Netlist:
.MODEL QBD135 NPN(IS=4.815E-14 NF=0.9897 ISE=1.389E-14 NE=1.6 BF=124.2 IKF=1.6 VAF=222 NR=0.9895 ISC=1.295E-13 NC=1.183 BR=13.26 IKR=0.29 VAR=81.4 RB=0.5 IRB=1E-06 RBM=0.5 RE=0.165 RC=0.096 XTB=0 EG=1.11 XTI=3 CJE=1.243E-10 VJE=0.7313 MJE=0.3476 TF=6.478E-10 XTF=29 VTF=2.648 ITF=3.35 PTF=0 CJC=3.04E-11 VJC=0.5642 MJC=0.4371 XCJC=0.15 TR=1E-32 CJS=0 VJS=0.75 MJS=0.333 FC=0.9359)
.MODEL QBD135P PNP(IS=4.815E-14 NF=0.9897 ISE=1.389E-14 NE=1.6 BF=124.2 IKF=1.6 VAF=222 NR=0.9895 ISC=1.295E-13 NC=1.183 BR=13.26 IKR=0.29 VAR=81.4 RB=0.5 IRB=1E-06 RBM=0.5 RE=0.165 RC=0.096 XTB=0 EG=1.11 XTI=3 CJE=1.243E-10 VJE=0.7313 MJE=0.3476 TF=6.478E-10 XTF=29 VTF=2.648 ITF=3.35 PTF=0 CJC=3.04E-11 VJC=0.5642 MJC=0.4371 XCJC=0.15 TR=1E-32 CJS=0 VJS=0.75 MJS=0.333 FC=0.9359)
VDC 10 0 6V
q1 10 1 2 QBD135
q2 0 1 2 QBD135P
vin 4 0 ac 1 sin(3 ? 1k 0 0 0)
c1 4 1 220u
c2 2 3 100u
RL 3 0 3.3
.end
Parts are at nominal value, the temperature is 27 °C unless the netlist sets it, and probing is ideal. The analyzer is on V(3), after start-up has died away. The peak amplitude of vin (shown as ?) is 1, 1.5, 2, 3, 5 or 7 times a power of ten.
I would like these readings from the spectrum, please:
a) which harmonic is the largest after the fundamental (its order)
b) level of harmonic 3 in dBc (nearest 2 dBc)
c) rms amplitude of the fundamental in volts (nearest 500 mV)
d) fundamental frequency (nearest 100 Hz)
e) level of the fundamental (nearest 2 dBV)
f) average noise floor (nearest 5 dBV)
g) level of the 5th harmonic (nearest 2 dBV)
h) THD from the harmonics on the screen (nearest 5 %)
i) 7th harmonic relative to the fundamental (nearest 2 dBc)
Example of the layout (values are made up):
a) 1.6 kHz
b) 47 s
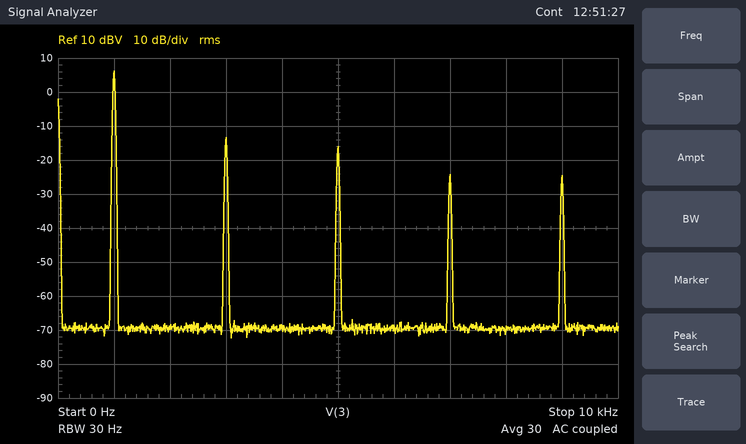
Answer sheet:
a) 3
b) -20 dBc
c) 2.0 V
d) 1.0 kHz
e) 6 dBV
f) -70 dBV
g) -16 dBV
h) 15 %
i) -30 dBc
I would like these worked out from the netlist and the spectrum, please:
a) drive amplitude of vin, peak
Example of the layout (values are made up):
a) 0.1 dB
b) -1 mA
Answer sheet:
a) 5 V
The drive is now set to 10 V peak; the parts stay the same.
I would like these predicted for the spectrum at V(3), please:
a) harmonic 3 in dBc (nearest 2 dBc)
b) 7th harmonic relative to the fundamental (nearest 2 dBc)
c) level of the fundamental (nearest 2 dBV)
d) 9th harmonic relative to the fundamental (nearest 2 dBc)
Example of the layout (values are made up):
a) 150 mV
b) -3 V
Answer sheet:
a) -14 dBc
b) -28 dBc
c) 8 dBV
d) -30 dBc
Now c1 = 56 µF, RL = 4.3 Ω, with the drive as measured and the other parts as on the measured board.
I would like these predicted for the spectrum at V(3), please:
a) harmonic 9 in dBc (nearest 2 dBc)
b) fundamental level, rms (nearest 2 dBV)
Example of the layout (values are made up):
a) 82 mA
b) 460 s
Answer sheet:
a) -36 dBc
b) 6 dBV
